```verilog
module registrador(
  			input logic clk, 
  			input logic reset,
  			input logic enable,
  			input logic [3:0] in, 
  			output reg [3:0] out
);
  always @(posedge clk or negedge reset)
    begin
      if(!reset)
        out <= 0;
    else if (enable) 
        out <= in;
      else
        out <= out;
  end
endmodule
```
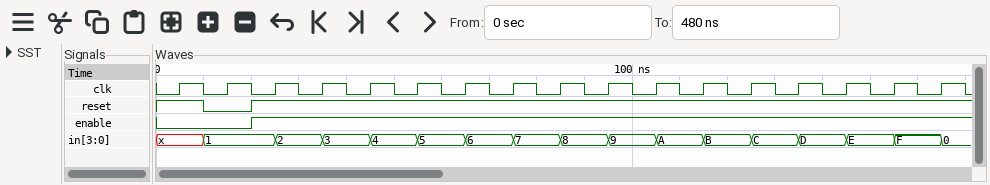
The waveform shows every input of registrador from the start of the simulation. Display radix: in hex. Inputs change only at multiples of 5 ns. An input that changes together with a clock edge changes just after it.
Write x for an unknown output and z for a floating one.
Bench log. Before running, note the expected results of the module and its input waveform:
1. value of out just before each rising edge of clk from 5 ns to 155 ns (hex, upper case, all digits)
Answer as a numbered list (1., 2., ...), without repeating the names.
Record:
1. x, 0, 0, 1, 2, 3, 4, 5, 6, 7, 8, 9, A, B, C, D
